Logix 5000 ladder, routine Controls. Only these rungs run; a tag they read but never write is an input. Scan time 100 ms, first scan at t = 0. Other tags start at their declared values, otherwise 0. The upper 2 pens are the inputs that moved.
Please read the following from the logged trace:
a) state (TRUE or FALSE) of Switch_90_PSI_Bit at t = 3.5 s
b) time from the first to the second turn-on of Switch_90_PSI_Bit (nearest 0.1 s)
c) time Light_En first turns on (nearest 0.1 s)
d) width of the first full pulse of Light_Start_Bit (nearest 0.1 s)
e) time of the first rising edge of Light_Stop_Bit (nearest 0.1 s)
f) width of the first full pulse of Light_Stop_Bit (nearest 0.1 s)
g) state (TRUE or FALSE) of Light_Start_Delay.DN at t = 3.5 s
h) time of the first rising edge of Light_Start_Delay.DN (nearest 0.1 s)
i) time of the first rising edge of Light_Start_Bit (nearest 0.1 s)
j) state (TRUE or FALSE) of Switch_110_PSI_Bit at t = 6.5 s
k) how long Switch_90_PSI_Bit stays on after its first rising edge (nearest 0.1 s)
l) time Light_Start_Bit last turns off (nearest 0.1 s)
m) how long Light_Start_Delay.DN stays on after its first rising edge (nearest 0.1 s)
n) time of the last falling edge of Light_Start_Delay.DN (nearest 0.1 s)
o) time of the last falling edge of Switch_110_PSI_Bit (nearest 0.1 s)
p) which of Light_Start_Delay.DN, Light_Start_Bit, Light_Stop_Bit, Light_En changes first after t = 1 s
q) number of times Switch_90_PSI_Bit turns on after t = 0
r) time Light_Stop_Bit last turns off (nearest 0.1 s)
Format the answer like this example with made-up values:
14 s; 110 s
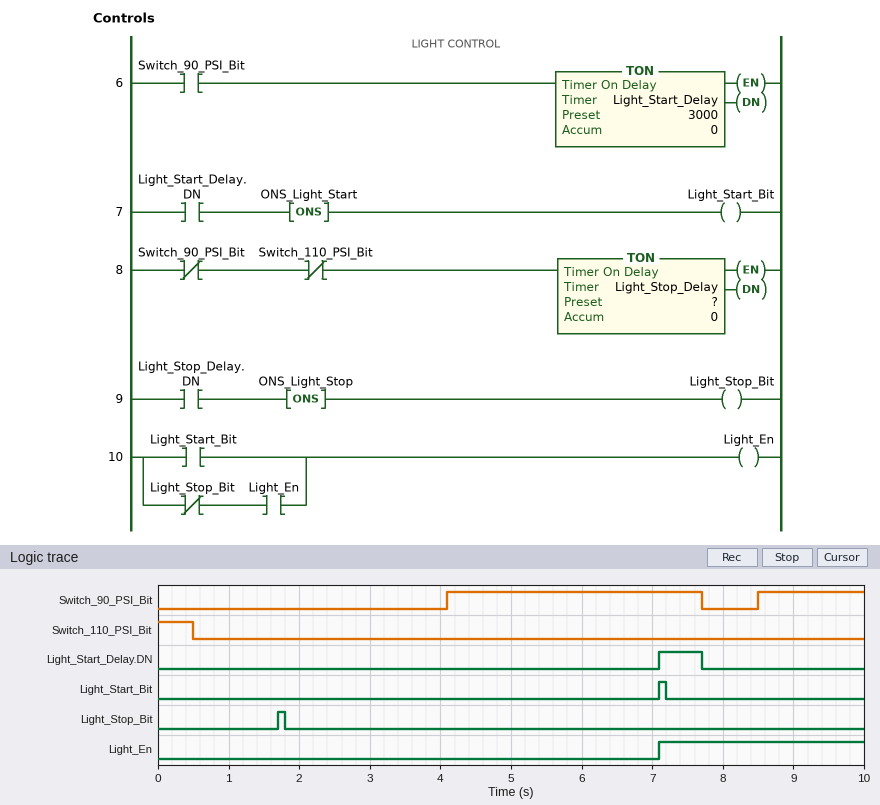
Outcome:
FALSE; 4.4 s; 7.1 s; 0.1 s; 1.7 s; 0.1 s; FALSE; 7.1 s; 7.1 s; FALSE; 3.6 s; 7.2 s; 0.6 s; 7.7 s; 0.5 s; Light_Stop_Bit; 2; 1.8 s
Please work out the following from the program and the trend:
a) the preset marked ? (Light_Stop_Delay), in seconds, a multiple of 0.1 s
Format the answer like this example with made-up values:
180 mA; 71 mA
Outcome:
1.2 s
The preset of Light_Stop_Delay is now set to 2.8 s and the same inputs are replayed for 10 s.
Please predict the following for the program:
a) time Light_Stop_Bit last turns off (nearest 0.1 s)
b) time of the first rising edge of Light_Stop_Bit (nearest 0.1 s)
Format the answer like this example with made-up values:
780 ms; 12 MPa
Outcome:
3.4 s; 3.3 s
